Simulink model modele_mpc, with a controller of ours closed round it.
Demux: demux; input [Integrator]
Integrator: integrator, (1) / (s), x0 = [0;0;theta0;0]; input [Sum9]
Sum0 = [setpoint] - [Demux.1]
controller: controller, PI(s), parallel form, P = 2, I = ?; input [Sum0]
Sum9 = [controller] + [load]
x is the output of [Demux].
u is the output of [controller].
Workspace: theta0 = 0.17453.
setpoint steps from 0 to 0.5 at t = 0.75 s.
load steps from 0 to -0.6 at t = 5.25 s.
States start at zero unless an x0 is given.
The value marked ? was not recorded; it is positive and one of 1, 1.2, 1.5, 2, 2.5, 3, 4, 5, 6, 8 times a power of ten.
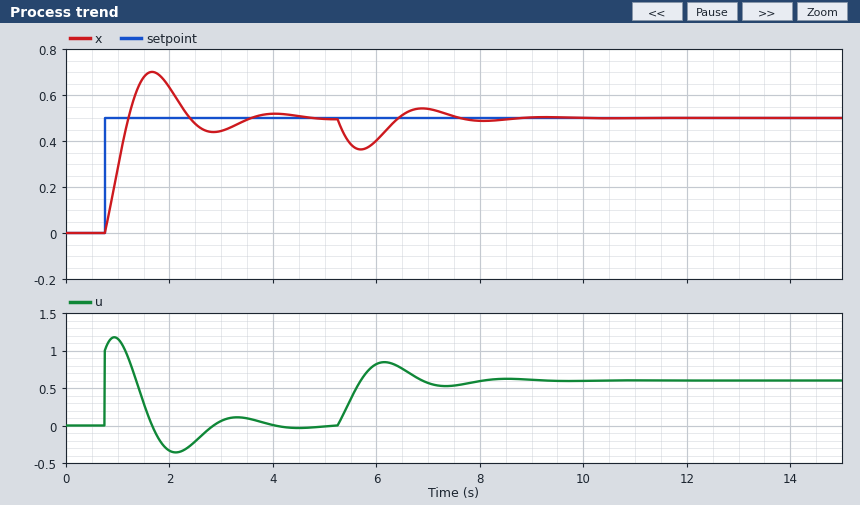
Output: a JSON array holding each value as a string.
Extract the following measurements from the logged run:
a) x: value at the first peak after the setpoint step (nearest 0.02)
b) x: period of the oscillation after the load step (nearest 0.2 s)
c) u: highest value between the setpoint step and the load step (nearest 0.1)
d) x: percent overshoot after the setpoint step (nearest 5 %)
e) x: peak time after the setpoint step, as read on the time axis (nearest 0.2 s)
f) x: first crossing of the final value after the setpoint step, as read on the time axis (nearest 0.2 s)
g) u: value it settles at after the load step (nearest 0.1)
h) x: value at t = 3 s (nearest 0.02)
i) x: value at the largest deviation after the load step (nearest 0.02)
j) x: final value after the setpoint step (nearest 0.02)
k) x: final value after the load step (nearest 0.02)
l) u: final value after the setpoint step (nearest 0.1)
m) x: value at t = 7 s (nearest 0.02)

["0.70", "2.4 s", "1.2", "40 %", "1.6 s", "1.2 s", "0.6", "0.44", "0.36", "0.50", "0.50", "0.0", "0.54"]
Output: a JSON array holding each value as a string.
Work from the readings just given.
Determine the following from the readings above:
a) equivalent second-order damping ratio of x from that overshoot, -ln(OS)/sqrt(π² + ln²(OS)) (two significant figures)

["0.28"]
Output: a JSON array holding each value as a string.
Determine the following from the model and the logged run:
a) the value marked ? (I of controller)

["8"]
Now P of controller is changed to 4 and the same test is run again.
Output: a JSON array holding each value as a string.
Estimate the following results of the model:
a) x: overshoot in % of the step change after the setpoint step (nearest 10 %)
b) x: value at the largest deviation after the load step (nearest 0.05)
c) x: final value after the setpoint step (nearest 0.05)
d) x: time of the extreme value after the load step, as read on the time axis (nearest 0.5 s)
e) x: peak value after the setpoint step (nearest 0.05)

["20 %", "0.40", "0.50", "5.5 s", "0.60"]
